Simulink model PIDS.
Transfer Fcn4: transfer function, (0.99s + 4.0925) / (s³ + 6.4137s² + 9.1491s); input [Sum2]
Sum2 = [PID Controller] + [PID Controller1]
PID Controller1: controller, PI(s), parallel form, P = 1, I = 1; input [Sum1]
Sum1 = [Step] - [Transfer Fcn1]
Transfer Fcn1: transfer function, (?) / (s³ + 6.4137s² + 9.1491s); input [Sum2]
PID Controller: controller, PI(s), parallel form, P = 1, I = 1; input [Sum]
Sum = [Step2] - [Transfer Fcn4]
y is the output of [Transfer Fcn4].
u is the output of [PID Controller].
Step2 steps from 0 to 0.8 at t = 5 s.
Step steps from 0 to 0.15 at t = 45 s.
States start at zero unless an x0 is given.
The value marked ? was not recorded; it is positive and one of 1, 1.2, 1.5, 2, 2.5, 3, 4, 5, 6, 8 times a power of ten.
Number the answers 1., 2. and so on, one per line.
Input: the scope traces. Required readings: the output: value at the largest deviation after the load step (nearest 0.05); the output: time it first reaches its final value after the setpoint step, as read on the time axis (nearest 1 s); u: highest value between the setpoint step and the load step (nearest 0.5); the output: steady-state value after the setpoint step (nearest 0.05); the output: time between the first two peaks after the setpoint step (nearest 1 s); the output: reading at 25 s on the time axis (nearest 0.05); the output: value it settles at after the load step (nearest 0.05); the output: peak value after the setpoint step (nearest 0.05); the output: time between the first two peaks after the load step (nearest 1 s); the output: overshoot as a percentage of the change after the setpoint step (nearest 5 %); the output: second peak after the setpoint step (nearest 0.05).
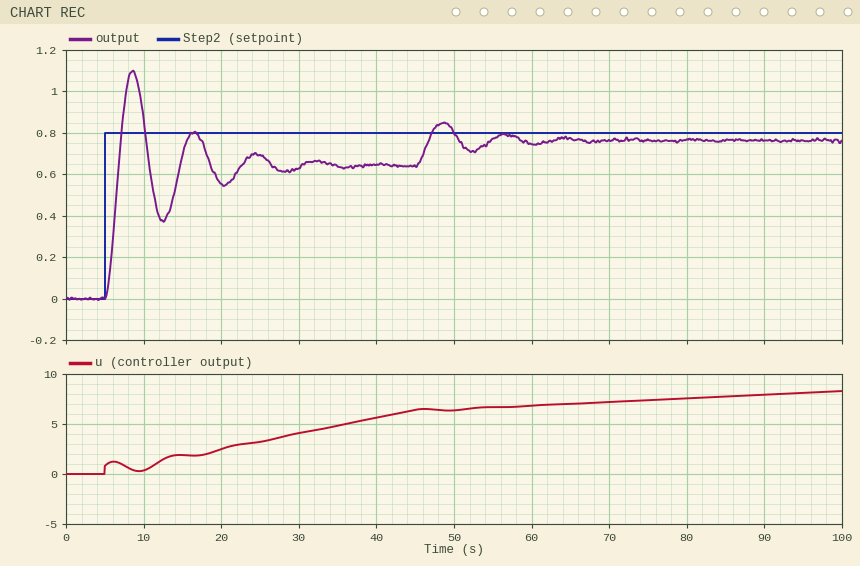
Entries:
1. 0.85
2. 7 s
3. 6.5
4. 0.65
5. 8 s
6. 0.70
7. 0.75
8. 1.10
9. 8 s
10. 70 %
11. 0.80
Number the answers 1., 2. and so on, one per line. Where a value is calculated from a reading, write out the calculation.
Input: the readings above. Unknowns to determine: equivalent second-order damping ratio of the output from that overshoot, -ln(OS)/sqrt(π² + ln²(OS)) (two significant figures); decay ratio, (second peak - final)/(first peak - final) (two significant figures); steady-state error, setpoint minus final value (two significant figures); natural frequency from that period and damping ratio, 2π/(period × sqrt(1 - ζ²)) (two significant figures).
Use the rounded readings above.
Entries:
1. ln(0.7) = -0.357; 0.357 / sqrt(9.870 + 0.127) = 0.11
2. (0.8 - 0.65) / (1.1 - 0.65) = 0.33
3. 0.8 - 0.65 = 0.15
4. 2π / (8 × sqrt(1 - 0.11²)) = 0.79 rad/s
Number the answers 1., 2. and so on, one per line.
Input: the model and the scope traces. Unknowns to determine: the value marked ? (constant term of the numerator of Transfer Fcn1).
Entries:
1. 1
